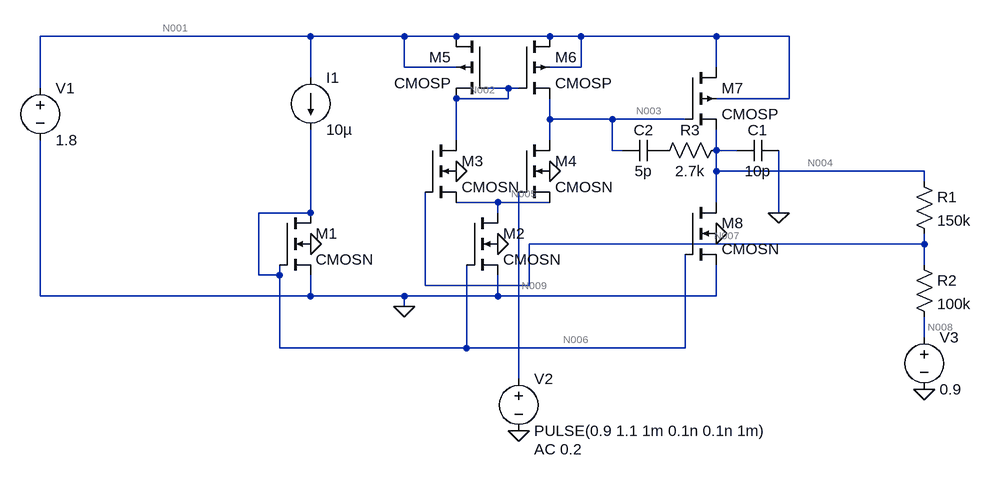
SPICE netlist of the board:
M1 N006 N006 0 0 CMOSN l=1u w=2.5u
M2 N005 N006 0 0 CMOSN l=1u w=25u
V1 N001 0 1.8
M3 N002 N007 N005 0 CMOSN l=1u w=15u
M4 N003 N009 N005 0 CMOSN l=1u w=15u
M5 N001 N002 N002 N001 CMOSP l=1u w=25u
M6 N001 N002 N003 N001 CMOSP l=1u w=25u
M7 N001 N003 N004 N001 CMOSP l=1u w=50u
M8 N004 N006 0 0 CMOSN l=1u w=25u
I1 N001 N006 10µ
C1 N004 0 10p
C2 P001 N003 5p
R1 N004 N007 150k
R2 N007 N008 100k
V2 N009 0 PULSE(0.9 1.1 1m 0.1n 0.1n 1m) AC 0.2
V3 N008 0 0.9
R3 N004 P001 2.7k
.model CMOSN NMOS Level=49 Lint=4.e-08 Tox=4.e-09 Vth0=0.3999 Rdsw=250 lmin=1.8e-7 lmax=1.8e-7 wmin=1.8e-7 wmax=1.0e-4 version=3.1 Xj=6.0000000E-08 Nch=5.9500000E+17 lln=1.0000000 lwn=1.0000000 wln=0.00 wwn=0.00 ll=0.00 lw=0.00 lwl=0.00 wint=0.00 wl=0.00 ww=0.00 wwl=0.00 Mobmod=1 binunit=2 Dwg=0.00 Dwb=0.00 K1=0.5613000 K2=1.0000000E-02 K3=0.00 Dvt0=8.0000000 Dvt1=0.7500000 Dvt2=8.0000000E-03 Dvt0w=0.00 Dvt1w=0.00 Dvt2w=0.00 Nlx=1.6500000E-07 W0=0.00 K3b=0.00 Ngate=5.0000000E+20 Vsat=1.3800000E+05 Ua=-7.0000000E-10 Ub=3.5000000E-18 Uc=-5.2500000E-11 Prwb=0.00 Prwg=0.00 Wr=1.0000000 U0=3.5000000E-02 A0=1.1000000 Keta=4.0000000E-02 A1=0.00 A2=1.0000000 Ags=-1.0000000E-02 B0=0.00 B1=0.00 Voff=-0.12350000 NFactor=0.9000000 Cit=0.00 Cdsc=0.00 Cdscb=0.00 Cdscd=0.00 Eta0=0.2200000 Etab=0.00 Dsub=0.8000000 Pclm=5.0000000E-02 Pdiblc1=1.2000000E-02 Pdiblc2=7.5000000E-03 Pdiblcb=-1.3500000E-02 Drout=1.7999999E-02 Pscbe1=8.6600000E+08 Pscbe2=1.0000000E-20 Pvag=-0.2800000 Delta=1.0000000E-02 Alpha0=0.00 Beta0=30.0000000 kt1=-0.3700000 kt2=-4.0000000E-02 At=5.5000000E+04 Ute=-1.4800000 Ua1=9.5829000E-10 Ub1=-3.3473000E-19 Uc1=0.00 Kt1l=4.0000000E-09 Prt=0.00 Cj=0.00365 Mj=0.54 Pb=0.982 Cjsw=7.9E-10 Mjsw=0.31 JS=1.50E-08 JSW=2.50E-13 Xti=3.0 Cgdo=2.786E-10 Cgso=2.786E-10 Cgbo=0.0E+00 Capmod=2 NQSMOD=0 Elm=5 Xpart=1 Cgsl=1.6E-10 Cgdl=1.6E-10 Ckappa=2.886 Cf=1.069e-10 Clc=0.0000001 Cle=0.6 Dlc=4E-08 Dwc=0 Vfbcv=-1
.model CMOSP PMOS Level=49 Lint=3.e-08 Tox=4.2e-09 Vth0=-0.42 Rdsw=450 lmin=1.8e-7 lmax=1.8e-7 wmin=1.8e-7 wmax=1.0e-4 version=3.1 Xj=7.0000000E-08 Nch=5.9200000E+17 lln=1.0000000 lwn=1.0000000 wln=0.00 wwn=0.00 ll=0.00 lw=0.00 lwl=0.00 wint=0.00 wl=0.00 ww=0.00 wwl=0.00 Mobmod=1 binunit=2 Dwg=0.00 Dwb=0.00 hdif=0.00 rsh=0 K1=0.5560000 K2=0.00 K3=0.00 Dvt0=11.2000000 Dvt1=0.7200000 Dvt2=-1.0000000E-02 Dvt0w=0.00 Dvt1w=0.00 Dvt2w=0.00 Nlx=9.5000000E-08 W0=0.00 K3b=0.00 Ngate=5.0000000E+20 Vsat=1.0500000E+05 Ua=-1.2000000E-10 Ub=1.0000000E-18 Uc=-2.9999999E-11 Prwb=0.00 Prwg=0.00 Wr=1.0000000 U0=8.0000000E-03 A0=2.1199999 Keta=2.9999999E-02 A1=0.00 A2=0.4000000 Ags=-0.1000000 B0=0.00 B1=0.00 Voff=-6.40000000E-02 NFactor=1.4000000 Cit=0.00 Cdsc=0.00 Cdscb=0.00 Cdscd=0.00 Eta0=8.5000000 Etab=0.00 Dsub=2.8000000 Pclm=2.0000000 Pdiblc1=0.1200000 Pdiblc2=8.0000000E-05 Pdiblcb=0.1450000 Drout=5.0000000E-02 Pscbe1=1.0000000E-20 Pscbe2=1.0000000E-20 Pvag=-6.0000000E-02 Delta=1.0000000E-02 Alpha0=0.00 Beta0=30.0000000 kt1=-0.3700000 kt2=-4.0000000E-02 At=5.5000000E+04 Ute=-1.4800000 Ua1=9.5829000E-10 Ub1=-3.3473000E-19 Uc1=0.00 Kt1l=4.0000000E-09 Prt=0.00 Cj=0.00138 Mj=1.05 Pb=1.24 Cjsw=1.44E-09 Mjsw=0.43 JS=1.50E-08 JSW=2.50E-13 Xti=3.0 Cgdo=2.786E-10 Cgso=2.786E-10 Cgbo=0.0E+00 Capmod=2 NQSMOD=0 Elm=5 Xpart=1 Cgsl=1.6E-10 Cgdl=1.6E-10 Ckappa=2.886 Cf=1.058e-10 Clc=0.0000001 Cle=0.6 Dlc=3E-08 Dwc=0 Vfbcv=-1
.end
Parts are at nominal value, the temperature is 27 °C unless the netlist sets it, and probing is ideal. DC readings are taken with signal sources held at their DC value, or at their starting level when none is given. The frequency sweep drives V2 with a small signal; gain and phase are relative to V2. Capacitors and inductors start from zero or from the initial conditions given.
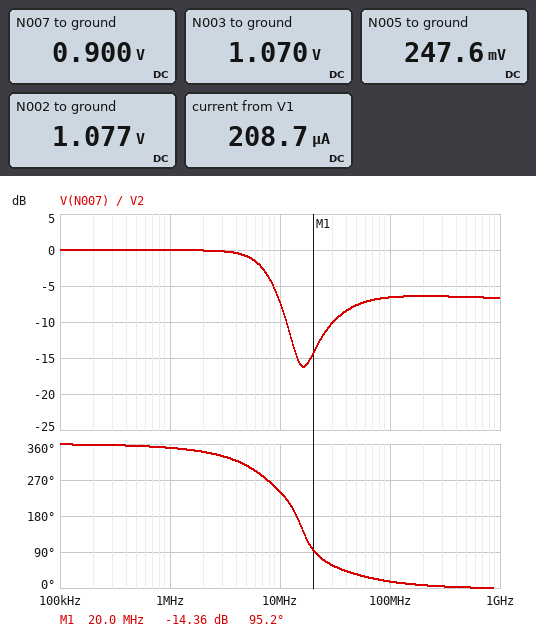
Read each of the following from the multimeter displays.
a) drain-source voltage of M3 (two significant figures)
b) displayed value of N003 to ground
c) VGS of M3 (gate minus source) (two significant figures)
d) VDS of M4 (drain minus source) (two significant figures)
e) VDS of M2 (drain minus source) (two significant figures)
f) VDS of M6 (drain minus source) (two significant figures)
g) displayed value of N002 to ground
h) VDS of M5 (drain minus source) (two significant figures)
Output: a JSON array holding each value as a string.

["830 mV", "1.070 V", "650 mV", "820 mV", "250 mV", "730 mV", "1.077 V", "720 mV"]
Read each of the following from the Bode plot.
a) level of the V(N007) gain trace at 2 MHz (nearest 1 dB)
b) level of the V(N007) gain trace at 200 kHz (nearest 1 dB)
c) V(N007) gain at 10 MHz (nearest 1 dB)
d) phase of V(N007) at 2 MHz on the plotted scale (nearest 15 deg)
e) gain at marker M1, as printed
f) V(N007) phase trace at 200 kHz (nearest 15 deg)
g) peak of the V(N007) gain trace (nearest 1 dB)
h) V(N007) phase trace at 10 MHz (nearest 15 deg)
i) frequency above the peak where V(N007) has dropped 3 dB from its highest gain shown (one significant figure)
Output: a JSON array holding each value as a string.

["0 dB", "0 dB", "-7 dB", "345 deg", "-14.36 dB", "360 deg", "0 dB", "240 deg", "7 MHz"]
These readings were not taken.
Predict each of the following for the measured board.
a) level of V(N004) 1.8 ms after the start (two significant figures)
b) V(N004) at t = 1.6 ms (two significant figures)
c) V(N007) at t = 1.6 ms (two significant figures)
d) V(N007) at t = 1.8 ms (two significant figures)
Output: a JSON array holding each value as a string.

["1.4 V", "1.4 V", "1.1 V", "1.1 V"]
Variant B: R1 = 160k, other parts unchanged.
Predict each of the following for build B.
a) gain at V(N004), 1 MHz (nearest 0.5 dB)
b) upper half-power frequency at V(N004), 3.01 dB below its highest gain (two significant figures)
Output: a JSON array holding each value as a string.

["8.5 dB", "8.4 MHz"]
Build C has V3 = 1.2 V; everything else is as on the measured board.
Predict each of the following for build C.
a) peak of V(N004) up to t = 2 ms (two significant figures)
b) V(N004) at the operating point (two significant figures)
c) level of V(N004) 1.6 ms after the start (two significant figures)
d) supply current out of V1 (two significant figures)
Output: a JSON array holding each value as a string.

["960 mV", "450 mV", "950 mV", "200 µA"]
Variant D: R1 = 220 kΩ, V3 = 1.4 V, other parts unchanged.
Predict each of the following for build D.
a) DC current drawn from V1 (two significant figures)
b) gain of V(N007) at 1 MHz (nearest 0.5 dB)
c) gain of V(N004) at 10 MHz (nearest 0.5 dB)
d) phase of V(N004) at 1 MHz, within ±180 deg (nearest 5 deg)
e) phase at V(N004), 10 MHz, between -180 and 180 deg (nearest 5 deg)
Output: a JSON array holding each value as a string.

["110 µA", "-43.5 dB", "-19.0 dB", "-105 deg", "165 deg"]
